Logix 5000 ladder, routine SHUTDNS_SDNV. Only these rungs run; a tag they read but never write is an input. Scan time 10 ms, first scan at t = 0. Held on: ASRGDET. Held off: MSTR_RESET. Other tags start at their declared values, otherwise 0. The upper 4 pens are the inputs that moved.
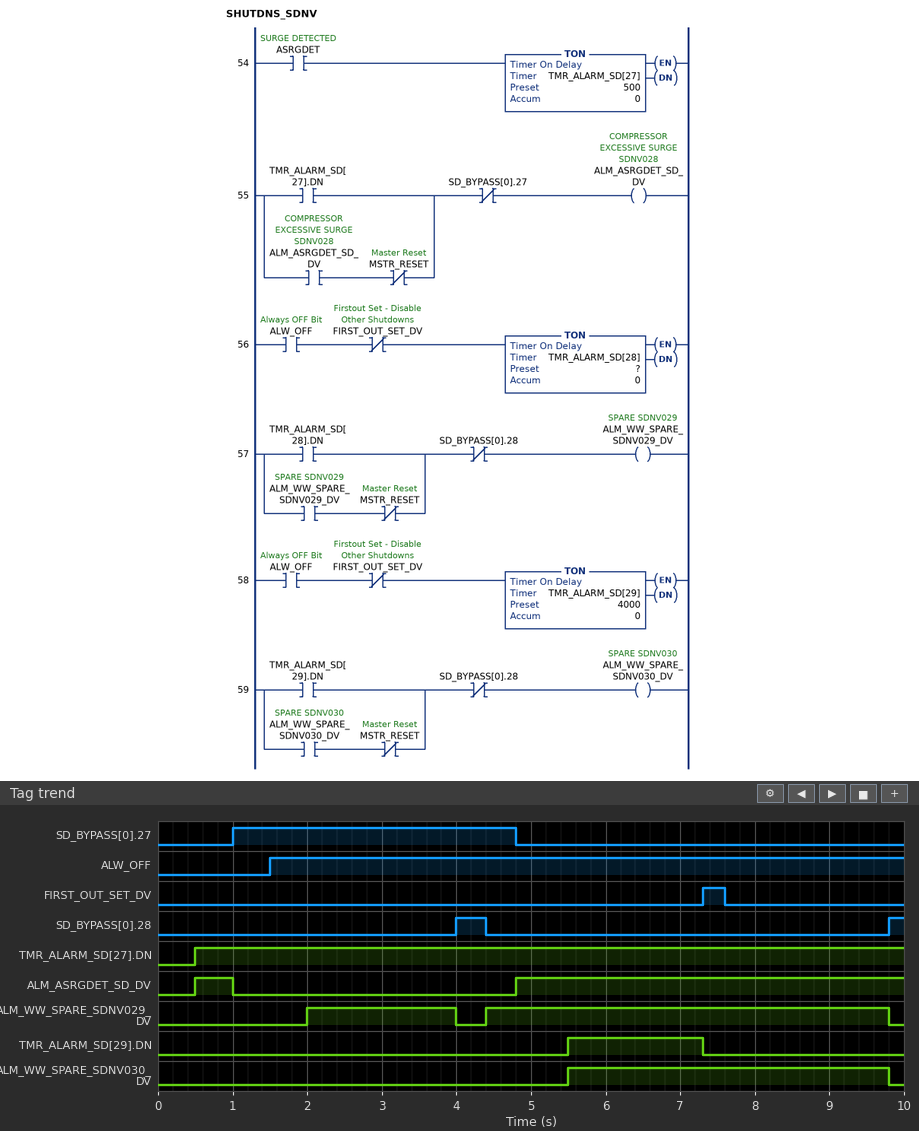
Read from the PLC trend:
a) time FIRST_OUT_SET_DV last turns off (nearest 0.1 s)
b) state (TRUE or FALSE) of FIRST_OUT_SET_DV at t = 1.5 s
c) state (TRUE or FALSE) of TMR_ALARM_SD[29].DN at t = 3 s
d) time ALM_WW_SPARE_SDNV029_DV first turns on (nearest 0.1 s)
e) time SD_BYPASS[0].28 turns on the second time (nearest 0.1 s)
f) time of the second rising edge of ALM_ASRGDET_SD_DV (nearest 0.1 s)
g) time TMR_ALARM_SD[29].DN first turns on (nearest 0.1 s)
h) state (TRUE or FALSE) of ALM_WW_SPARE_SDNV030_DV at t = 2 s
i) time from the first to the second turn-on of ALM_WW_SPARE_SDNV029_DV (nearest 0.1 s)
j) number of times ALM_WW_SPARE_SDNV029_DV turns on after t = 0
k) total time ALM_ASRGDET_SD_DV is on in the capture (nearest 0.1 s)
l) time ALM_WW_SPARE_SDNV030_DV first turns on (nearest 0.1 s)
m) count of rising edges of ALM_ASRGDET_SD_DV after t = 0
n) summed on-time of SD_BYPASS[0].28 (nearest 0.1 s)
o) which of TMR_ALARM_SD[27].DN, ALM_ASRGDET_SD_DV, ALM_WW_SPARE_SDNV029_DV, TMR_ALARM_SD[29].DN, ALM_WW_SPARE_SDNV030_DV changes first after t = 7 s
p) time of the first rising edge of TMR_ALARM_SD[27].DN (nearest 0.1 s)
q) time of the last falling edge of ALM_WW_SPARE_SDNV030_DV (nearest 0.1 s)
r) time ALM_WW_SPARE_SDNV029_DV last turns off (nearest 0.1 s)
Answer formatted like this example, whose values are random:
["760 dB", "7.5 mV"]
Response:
["7.6 s", "FALSE", "FALSE", "2.0 s", "9.8 s", "4.8 s", "5.5 s", "FALSE", "2.4 s", "2", "5.7 s", "5.5 s", "2", "0.6 s", "TMR_ALARM_SD[29].DN", "0.5 s", "9.8 s", "9.8 s"]
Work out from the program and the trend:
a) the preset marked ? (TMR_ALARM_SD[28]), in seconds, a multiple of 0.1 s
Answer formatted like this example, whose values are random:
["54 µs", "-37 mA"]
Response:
["0.5 s"]
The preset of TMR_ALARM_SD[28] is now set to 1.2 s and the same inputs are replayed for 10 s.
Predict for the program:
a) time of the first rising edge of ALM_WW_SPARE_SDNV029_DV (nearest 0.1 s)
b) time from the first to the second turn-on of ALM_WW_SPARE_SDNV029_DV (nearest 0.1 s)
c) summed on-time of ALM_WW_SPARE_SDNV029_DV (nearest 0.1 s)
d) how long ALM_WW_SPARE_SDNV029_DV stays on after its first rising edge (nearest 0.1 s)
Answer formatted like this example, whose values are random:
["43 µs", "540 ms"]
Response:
["2.7 s", "1.7 s", "6.7 s", "1.3 s"]
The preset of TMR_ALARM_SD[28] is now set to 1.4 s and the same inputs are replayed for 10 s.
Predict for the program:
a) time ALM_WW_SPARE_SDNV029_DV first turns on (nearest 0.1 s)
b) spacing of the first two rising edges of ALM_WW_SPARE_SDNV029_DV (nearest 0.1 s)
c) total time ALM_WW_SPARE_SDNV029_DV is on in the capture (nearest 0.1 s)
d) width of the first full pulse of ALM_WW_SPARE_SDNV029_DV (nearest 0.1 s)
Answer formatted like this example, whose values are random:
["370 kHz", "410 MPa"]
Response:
["2.9 s", "1.5 s", "6.5 s", "1.1 s"]
